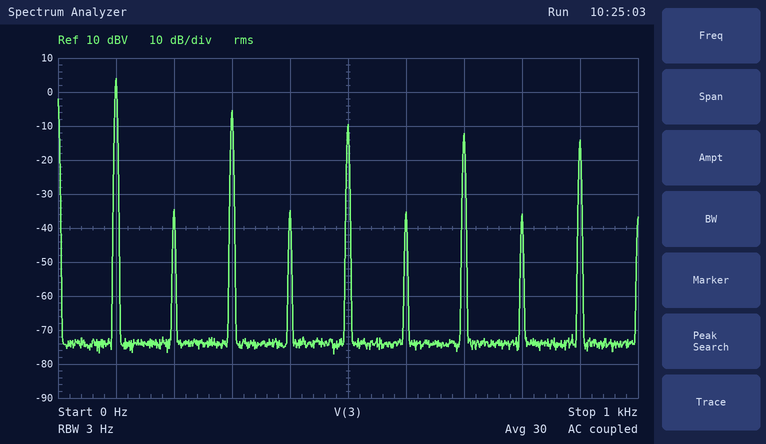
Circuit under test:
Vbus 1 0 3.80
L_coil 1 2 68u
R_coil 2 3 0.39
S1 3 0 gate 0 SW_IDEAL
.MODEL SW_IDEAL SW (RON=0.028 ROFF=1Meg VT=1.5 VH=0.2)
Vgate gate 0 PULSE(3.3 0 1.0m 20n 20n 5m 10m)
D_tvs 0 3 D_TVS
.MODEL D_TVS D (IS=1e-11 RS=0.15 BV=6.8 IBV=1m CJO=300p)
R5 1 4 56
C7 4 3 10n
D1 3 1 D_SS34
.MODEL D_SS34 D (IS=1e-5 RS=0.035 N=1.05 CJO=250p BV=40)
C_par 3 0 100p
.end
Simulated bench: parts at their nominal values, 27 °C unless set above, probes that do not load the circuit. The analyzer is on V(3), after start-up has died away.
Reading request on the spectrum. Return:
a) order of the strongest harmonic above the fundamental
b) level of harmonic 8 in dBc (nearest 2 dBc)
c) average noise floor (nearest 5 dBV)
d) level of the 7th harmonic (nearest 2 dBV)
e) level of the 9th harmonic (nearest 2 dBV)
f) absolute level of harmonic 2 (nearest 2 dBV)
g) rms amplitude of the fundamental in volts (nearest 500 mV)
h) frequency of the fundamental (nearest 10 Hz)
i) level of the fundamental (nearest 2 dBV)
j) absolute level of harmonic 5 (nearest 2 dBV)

3
-40 dBc
-75 dBV
-12 dBV
-14 dBV
-34 dBV
1.5 V
100 Hz
4 dBV
-10 dBV
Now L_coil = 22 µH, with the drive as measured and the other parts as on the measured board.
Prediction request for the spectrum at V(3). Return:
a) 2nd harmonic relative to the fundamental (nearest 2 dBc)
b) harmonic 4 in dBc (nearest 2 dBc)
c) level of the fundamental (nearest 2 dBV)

-48 dBc
-48 dBc
4 dBV
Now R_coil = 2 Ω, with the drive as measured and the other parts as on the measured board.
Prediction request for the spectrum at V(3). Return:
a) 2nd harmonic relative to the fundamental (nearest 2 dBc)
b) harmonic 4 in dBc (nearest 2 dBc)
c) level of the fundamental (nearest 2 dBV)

-54 dBc
-54 dBc
4 dBV
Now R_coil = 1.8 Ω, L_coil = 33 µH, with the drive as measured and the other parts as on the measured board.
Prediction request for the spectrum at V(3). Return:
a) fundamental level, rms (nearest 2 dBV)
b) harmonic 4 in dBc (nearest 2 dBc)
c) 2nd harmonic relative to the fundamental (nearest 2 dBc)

4 dBV
-58 dBc
-58 dBc
